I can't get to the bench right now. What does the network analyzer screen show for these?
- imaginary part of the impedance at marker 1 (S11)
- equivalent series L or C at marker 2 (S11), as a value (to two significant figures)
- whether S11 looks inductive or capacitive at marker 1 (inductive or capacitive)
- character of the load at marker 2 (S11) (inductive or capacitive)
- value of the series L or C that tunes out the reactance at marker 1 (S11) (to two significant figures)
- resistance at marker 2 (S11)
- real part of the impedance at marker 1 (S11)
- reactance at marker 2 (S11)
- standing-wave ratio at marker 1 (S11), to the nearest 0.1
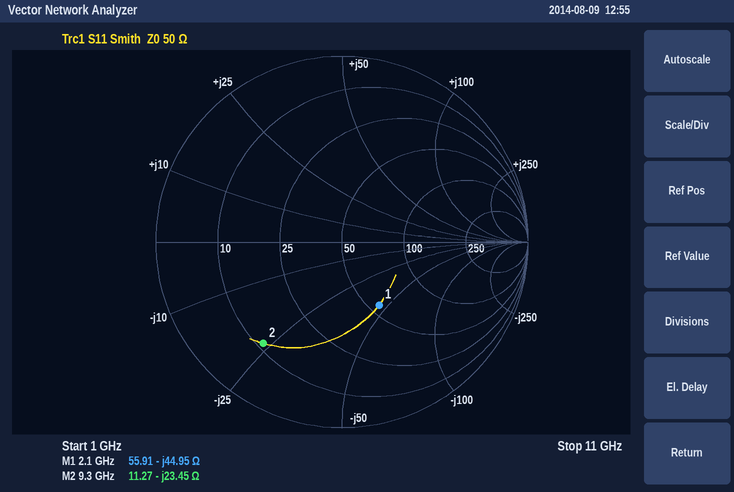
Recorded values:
-44.95 Ω
730 fF
capacitive
capacitive
3.4 nH
11.27 Ω
55.91 Ω
-23.45 Ω
2.3
